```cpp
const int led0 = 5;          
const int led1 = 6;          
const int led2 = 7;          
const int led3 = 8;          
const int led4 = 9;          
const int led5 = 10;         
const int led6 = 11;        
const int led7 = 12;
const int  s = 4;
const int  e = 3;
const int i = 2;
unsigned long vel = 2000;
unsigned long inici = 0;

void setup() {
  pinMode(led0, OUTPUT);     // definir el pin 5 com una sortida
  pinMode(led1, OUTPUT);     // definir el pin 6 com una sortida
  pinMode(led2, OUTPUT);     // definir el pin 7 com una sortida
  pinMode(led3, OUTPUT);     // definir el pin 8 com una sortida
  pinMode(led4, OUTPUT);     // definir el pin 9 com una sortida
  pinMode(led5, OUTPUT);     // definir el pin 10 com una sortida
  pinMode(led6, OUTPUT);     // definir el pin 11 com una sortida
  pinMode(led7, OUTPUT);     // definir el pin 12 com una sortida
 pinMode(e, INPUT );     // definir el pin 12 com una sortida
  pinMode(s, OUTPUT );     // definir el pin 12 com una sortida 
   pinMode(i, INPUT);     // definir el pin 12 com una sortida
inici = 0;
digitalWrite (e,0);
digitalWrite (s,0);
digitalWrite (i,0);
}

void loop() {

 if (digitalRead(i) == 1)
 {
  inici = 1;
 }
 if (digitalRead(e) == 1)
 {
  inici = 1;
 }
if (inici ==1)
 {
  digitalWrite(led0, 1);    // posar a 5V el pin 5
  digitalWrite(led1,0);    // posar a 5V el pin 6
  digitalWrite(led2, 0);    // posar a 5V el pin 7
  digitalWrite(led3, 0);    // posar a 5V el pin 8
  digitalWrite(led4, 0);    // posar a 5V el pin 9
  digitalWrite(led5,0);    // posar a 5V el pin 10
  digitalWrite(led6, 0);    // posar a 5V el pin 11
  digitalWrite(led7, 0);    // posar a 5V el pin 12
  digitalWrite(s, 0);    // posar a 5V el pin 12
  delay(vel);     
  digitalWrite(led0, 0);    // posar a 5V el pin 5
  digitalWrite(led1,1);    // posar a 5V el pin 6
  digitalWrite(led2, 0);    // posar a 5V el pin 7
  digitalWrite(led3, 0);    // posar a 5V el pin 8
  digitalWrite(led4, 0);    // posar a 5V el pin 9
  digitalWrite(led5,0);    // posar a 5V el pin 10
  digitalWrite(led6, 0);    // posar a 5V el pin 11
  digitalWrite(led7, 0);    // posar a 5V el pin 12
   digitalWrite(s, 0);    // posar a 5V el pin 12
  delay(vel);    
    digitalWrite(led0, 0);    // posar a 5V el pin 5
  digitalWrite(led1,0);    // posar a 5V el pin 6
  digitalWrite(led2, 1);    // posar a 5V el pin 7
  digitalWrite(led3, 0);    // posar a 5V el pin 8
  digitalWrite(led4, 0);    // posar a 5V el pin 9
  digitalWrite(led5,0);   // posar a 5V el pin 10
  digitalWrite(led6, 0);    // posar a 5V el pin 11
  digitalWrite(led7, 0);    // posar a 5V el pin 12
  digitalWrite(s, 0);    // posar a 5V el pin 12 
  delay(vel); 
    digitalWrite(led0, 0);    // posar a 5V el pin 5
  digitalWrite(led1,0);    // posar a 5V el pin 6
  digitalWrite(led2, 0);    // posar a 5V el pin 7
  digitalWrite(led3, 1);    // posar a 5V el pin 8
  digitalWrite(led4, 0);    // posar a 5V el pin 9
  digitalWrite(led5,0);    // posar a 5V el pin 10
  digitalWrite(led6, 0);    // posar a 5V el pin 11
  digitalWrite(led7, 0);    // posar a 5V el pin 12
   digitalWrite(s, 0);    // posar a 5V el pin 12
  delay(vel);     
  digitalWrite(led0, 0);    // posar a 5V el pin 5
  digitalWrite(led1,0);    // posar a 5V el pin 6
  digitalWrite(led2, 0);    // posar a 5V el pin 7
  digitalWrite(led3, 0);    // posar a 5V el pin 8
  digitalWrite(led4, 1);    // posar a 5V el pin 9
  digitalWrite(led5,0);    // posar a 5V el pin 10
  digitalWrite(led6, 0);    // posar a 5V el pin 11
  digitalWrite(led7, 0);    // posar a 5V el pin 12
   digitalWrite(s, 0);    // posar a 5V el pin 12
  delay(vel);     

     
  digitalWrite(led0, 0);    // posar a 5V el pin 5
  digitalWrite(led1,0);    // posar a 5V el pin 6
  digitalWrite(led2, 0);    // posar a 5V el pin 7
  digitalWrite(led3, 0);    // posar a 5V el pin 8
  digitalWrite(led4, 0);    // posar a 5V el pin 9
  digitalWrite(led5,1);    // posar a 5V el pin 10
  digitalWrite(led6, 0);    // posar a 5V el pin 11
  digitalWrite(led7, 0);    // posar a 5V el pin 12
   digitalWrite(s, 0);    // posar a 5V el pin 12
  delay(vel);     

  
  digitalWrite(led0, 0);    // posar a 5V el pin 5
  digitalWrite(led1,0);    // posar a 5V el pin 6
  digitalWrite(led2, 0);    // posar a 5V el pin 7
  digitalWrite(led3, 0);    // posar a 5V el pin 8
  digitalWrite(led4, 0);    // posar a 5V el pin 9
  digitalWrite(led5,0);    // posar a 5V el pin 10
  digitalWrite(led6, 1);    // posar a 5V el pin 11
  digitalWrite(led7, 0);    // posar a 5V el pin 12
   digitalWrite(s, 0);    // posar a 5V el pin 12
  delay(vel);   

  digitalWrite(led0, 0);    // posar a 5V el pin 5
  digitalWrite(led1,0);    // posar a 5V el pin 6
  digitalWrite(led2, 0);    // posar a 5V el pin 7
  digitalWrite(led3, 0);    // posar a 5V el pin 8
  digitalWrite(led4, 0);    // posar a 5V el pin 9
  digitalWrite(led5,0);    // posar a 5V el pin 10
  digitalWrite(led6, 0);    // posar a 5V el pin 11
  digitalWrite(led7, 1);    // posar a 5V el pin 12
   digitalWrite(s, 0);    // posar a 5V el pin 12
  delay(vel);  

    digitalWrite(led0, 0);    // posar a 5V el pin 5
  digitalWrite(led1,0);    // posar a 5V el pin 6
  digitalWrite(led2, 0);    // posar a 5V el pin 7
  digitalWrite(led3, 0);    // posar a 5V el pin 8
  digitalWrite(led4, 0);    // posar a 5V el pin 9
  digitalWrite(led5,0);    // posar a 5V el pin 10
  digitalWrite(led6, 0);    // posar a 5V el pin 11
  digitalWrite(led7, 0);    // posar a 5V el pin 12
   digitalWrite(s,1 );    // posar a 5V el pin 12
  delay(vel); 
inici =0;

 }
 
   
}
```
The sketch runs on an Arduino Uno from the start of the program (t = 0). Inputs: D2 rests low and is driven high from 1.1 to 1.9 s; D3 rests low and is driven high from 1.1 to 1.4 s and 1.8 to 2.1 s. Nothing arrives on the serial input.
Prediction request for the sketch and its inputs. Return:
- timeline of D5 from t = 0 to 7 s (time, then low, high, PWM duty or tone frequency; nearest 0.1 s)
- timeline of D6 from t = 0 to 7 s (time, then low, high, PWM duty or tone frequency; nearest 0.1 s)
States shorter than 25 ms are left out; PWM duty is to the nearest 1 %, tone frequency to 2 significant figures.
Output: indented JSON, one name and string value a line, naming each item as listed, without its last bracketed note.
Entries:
{
  "timeline of D5 from t = 0 to 7 s": "0 s low; 1.1 s high; 3.1 s low",
  "timeline of D6 from t = 0 to 7 s": "0 s low; 3.1 s high; 5.1 s low"
}
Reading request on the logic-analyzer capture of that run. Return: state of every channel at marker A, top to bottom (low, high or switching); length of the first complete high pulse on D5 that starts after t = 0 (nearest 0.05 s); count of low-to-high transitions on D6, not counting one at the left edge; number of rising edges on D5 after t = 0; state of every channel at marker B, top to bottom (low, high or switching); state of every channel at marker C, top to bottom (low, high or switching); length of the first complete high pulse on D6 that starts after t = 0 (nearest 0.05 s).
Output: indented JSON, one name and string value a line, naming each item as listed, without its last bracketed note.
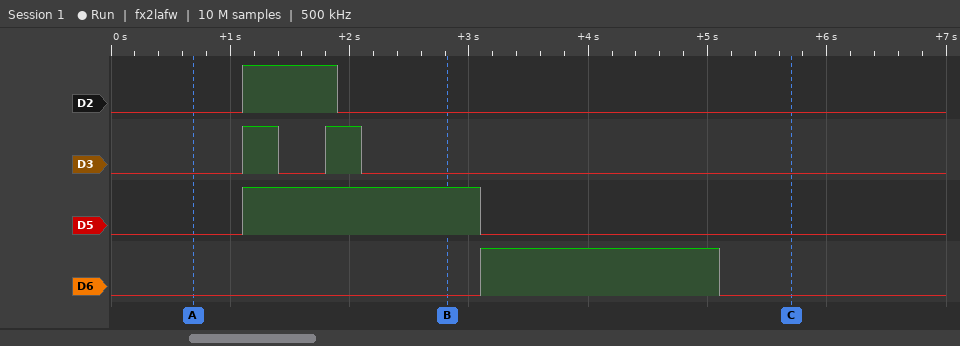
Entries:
{
  "state of every channel at marker A, top to bottom": "D2 low, D3 low, D5 low, D6 low",
  "length of the first complete high pulse on D5 that starts after t = 0": "2.00 s",
  "count of low-to-high transitions on D6, not counting one at the left edge": "1",
  "number of rising edges on D5 after t = 0": "1",
  "state of every channel at marker B, top to bottom": "D2 low, D3 low, D5 high, D6 low",
  "state of every channel at marker C, top to bottom": "D2 low, D3 low, D5 low, D6 low",
  "length of the first complete high pulse on D6 that starts after t = 0": "2.00 s"
}
